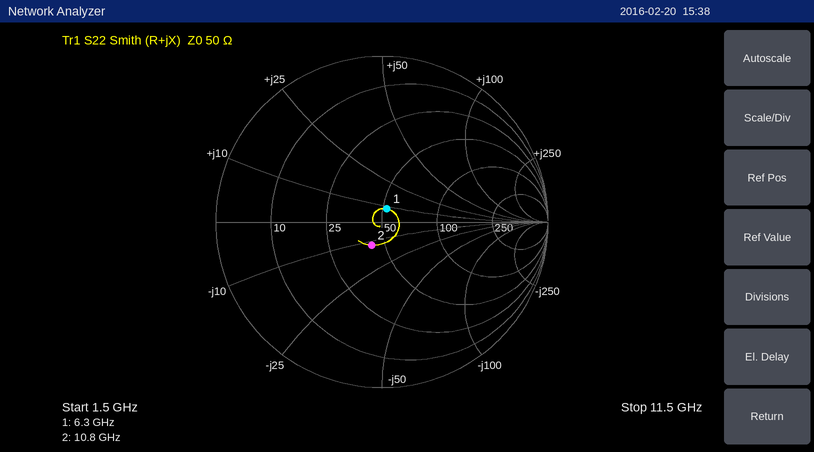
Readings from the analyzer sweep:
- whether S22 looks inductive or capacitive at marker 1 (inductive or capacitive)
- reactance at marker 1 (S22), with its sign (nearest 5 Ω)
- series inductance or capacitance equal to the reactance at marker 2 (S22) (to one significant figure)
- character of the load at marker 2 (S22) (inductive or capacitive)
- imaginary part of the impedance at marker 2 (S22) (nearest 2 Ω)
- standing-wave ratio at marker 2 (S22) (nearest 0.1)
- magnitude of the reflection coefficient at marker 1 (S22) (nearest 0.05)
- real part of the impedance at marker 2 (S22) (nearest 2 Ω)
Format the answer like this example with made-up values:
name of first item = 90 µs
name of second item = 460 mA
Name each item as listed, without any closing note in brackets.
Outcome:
whether S22 looks inductive or capacitive at marker 1 = inductive
reactance at marker 1 (S22), with its sign = +10 Ω
series inductance or capacitance equal to the reactance at marker 2 (S22) = 1 pF
character of the load at marker 2 (S22) = capacitive
imaginary part of the impedance at marker 2 (S22) = -12 Ω
standing-wave ratio at marker 2 (S22) = 1.4
magnitude of the reflection coefficient at marker 1 (S22) = 0.10
real part of the impedance at marker 2 (S22) = 42 Ω
